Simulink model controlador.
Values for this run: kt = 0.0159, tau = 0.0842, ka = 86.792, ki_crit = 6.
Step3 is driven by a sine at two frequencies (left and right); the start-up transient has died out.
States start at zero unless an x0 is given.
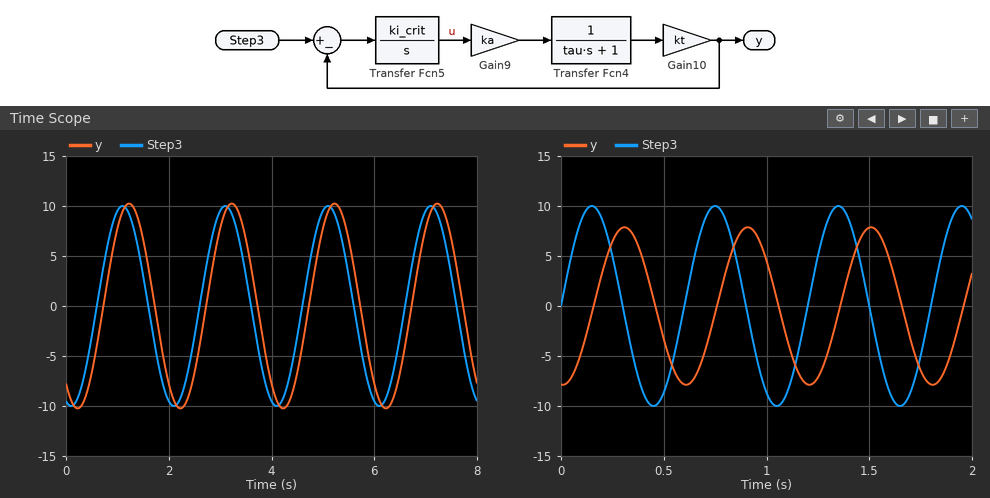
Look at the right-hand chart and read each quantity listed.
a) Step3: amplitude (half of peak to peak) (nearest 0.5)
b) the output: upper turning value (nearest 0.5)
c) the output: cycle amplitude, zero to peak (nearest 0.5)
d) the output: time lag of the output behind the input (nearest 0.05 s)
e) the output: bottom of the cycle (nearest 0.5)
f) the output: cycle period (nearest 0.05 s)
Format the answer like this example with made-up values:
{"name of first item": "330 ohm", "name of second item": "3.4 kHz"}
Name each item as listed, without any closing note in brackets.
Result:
{"Step3: amplitude (half of peak to peak)": "10.0", "the output: upper turning value": "8.0", "the output: cycle amplitude, zero to peak": "8.0", "the output: time lag of the output behind the input": "0.15 s", "the output: bottom of the cycle": "-8.0", "the output: cycle period": "0.60 s"}
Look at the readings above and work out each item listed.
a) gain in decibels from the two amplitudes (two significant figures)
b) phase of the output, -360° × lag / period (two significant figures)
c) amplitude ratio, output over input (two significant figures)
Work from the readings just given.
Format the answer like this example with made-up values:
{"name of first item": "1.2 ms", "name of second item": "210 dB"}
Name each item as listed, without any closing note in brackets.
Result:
{"gain in decibels from the two amplitudes": "-1.9 dB", "phase of the output, -360° × lag / period": "-90°", "amplitude ratio, output over input": "0.80"}
